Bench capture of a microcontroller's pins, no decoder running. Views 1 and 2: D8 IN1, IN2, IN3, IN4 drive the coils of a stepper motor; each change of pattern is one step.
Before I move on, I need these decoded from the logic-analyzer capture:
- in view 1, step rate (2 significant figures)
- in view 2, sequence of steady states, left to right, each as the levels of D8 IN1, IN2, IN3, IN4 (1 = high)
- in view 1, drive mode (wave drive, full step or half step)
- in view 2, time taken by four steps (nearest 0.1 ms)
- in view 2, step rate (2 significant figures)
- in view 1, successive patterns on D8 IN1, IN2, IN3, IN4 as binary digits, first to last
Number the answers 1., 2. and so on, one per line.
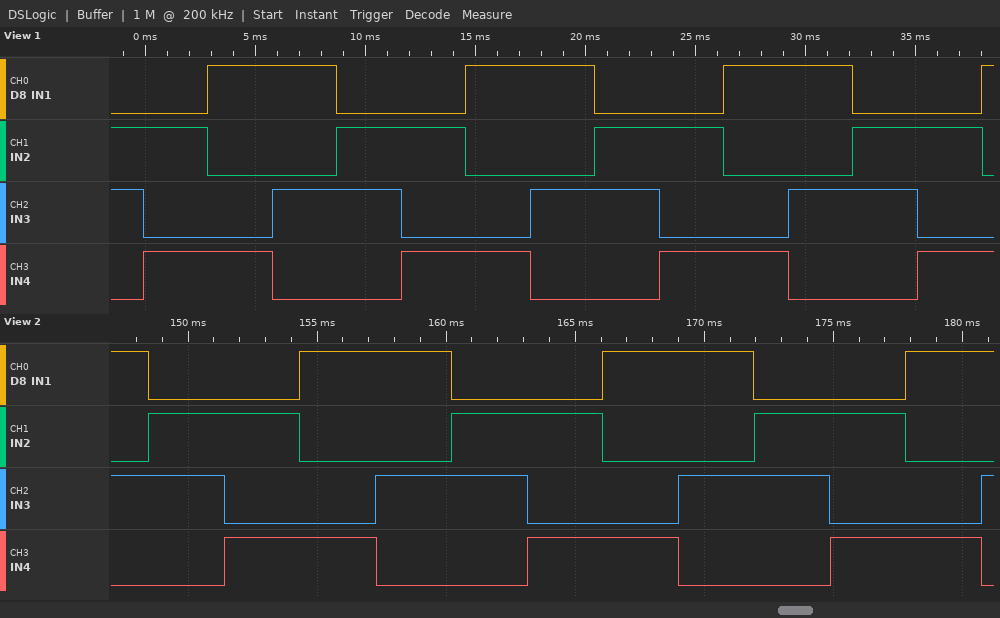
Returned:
1. 340 steps/s
2. 1010 0110 0101 1001 1010 0110 0101 1001 1010 0110 0101 1001 1010
3. full step
4. 11.7 ms
5. 340 steps/s
6. 0110 0101 1001 1010 0110 0101 1001 1010 0110 0101 1001 1010 0110 0101 1001
